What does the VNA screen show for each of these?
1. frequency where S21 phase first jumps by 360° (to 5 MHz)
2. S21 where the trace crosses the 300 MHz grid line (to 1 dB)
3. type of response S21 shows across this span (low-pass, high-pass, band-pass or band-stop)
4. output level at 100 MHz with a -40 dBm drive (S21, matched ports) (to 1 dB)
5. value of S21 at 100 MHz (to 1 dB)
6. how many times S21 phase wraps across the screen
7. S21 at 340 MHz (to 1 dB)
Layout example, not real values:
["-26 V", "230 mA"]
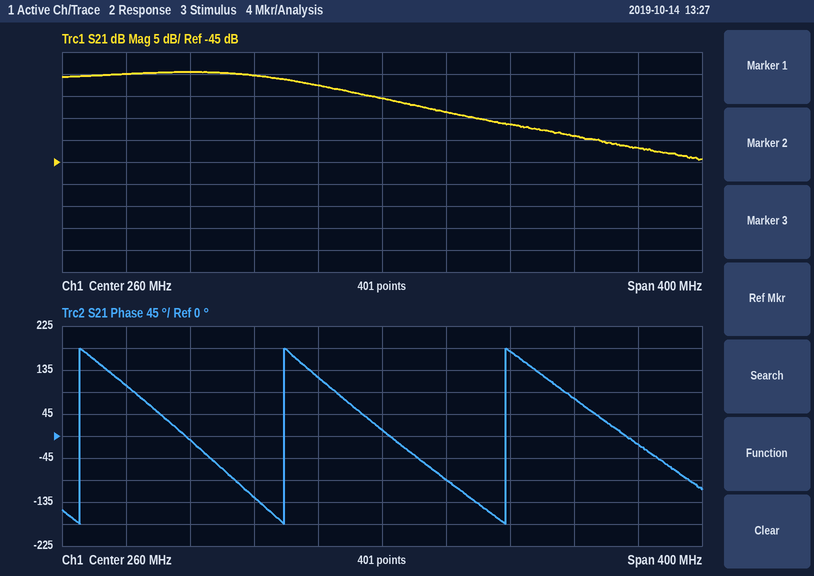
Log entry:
["70 MHz", "-34 dB", "low-pass", "-65 dBm", "-25 dB", "3", "-36 dB"]
